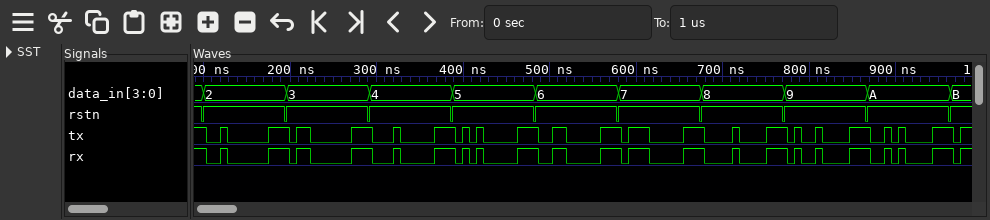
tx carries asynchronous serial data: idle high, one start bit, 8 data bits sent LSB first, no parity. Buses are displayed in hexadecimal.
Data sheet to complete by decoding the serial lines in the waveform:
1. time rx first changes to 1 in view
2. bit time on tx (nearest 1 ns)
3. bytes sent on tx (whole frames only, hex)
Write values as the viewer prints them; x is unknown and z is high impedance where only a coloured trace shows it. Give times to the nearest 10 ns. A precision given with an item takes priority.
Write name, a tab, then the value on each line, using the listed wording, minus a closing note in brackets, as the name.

time rx first changes to 1 in view	120 ns
bit time on tx	8 ns
bytes sent on tx	02, 03, 04, 05, 06, 07, 08, 09, 0A
